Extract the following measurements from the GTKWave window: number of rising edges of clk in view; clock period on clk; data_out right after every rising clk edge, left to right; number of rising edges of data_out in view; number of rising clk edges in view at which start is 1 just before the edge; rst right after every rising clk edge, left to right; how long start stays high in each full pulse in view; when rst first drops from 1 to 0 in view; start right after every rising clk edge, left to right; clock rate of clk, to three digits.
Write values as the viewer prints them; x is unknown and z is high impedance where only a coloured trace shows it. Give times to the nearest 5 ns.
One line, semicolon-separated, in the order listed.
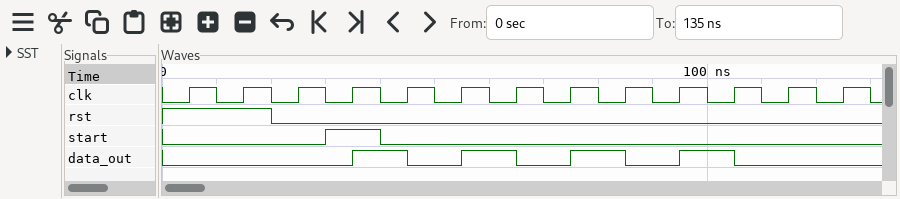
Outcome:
13; 10 ns; 0 0 0 1 0 1 0 1 0 1 0 0 0; 4; 1; 1 1 0 0 0 0 0 0 0 0 0 0 0; 10 ns; 20 ns; 0 0 0 1 0 0 0 0 0 0 0 0 0; 100 MHz
